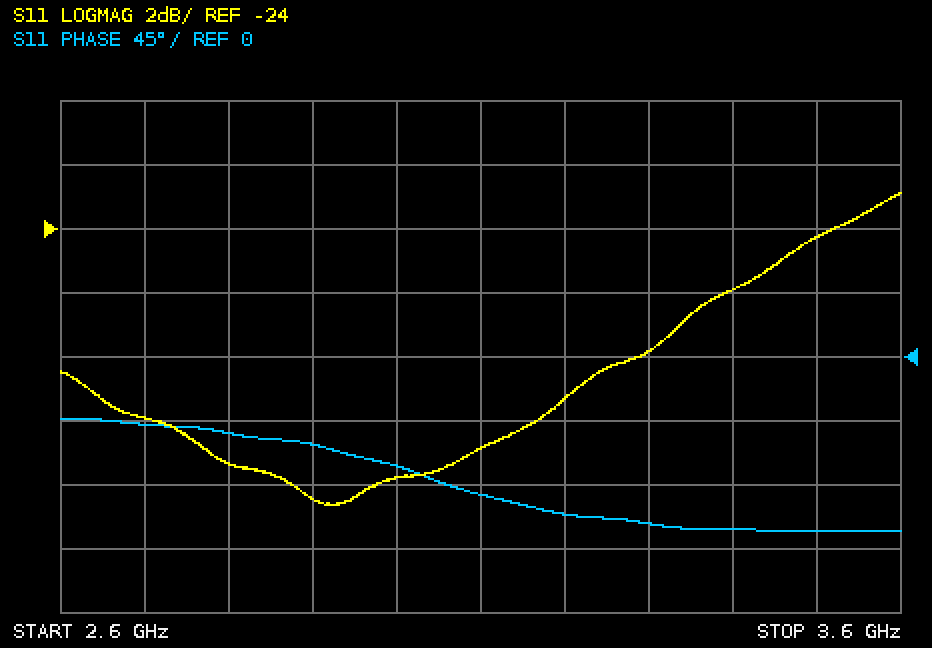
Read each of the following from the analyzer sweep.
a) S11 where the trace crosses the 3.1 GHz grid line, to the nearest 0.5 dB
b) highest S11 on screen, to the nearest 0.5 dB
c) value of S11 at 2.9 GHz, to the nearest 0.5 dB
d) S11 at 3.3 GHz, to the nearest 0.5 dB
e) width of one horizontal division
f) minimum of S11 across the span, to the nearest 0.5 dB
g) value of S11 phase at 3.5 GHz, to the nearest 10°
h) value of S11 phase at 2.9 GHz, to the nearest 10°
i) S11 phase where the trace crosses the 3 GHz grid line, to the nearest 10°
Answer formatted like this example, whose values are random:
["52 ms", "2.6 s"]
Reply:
["-31.0 dB", "-23.0 dB", "-32.5 dB", "-28.0 dB", "100 MHz", "-32.5 dB", "-120°", "-60°", "-80°"]
